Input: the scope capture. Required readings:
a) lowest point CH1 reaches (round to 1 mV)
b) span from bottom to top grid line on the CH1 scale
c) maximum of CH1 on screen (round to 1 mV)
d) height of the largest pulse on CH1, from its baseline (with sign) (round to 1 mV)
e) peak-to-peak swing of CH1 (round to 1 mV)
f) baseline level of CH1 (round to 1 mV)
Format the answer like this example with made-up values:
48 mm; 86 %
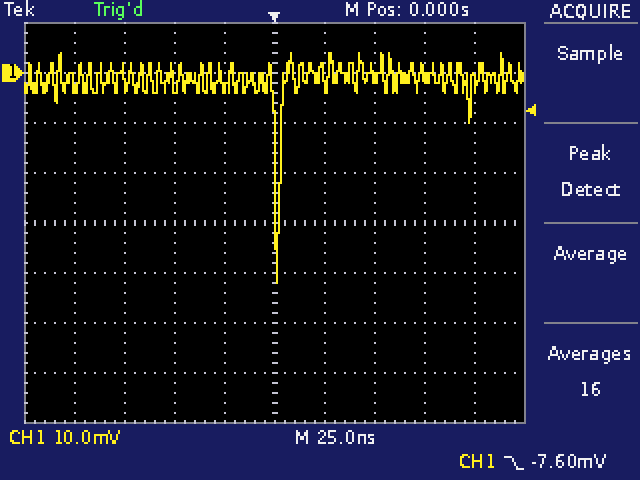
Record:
-42 mV; 80 mV; 4 mV; -41 mV; 46 mV; -1 mV
